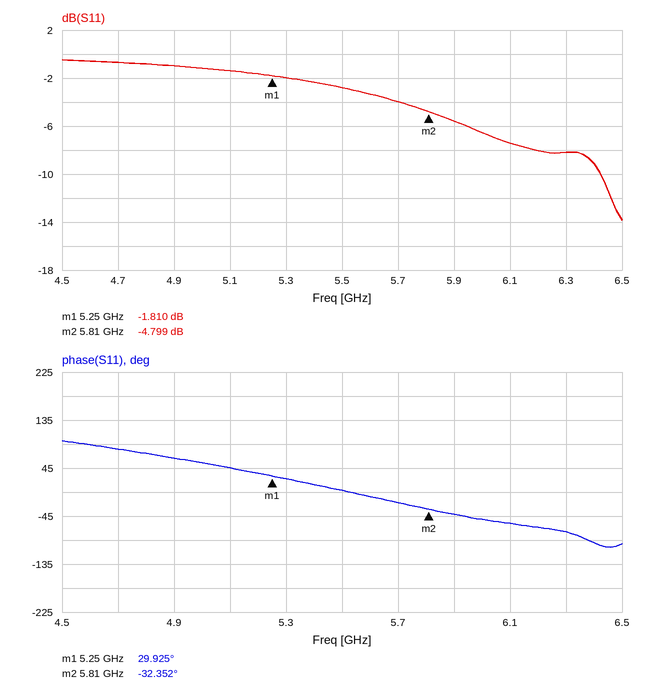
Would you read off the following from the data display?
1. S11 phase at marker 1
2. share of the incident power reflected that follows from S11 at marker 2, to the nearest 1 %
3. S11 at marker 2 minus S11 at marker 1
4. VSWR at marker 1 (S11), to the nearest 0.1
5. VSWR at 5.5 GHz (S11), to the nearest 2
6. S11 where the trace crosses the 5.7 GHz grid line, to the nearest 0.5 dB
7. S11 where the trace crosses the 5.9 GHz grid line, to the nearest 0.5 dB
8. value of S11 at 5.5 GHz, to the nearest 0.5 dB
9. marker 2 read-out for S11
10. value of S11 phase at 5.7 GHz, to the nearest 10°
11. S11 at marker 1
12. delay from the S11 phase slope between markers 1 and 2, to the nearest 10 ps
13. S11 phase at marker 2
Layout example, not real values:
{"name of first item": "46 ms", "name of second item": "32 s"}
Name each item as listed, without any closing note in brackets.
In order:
{"S11 phase at marker 1": "29.925°", "share of the incident power reflected that follows from S11 at marker 2, to the nearest 1 %": "33 %", "S11 at marker 2 minus S11 at marker 1": "-2.989 dB", "VSWR at marker 1 (S11), to the nearest 0.1": "9.6", "VSWR at 5.5 GHz (S11), to the nearest 2": "6", "S11 where the trace crosses the 5.7 GHz grid line, to the nearest 0.5 dB": "-4.0 dB", "S11 where the trace crosses the 5.9 GHz grid line, to the nearest 0.5 dB": "-5.5 dB", "value of S11 at 5.5 GHz, to the nearest 0.5 dB": "-3.0 dB", "marker 2 read-out for S11": "-4.799 dB", "value of S11 phase at 5.7 GHz, to the nearest 10°": "-20°", "S11 at marker 1": "-1.810 dB", "delay from the S11 phase slope between markers 1 and 2, to the nearest 10 ps": "310 ps", "S11 phase at marker 2": "-32.352°"}
